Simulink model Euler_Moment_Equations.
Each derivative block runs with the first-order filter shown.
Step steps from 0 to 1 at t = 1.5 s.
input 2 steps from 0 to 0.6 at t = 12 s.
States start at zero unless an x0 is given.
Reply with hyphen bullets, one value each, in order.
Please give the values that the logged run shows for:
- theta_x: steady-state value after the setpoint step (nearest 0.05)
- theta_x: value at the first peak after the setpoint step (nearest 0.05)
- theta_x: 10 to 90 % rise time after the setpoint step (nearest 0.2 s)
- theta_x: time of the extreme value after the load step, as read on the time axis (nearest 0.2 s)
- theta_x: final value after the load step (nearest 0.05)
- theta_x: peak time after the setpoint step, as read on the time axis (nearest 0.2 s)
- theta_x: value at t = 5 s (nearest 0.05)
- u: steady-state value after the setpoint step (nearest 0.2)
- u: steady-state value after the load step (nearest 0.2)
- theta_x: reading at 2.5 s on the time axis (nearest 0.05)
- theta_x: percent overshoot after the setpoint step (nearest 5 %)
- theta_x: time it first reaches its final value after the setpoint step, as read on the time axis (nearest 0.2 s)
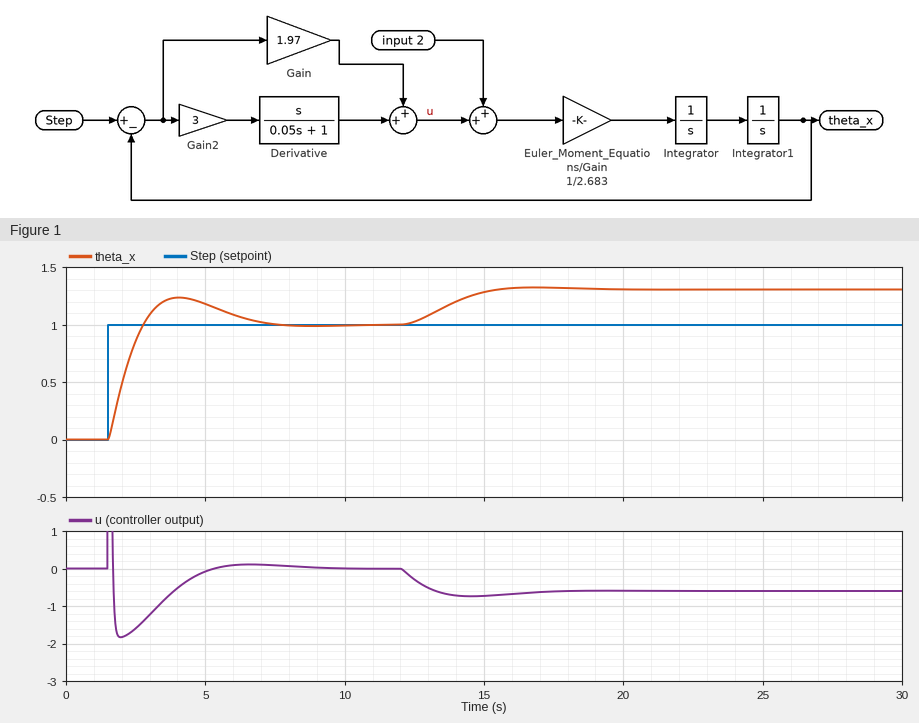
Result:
- 1.00
- 1.25
- 1.0 s
- 16.8 s
- 1.30
- 4.0 s
- 1.20
- 0.0
- -0.6
- 0.85
- 25 %
- 2.8 s
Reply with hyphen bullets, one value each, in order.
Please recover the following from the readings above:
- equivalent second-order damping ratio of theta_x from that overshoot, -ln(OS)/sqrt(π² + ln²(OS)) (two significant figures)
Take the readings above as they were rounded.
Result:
- 0.40
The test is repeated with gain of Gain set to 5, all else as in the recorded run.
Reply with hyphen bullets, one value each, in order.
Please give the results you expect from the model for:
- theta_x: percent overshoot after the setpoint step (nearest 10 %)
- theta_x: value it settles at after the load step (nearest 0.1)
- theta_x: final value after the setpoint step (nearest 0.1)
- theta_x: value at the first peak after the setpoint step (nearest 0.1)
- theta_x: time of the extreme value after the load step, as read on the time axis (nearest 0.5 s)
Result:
- 40 %
- 1.1
- 1.0
- 1.4
- 14.5 s
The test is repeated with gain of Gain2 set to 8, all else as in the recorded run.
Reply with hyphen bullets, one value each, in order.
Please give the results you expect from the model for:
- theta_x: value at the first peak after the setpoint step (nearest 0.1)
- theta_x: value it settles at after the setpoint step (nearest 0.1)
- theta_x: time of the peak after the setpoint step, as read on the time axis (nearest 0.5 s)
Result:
- 1.1
- 1.0
- 3.0 s
